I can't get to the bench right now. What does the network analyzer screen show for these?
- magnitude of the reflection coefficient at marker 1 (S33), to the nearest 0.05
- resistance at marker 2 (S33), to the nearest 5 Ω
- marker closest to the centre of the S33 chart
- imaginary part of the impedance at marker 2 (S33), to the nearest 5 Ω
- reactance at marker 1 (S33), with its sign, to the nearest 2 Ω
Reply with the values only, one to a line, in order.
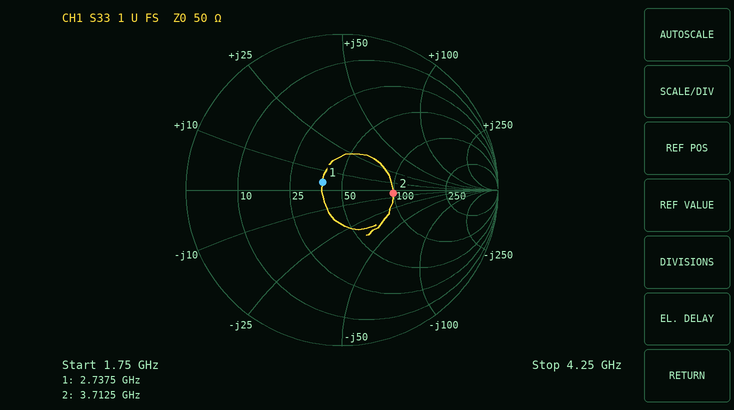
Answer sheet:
0.15
100 Ω
marker 1
-5 Ω
+4 Ω
